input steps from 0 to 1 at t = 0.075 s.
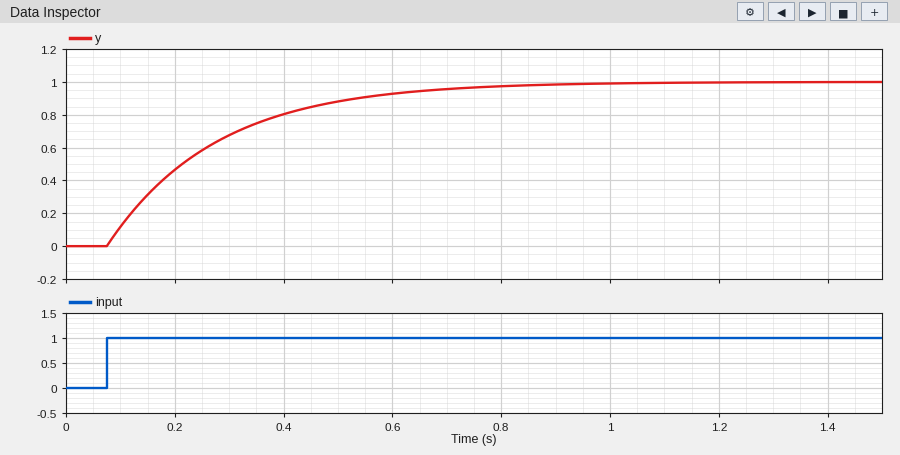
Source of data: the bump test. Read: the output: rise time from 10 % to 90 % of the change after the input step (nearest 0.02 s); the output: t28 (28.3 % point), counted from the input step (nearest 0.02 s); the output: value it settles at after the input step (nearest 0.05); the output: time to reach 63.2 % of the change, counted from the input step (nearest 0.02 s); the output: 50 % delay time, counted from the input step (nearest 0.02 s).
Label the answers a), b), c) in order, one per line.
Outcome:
a) 0.44 s
b) 0.06 s
c) 1.00
d) 0.20 s
e) 0.14 s
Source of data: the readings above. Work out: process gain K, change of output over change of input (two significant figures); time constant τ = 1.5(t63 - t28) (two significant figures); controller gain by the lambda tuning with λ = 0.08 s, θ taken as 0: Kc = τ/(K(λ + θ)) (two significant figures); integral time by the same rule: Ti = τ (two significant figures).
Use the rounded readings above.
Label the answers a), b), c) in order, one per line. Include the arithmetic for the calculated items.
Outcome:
a) (1 - 0) / 1 = 1.0
b) 1.5 × (0.2 - 0.06) = 0.21 s
c) 0.21 / (1 × (0.08 + 0)) = 2.6
d) 0.21 s
